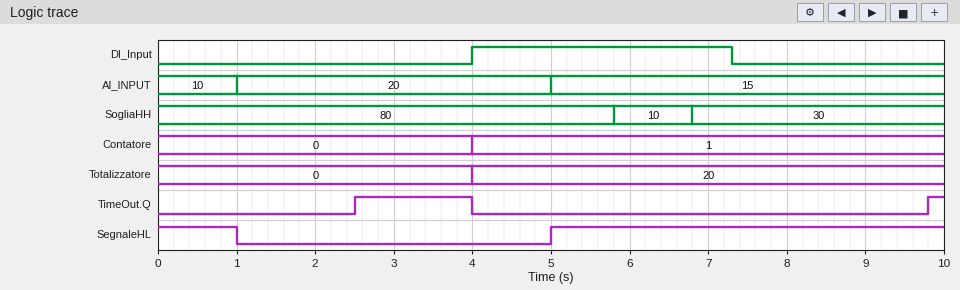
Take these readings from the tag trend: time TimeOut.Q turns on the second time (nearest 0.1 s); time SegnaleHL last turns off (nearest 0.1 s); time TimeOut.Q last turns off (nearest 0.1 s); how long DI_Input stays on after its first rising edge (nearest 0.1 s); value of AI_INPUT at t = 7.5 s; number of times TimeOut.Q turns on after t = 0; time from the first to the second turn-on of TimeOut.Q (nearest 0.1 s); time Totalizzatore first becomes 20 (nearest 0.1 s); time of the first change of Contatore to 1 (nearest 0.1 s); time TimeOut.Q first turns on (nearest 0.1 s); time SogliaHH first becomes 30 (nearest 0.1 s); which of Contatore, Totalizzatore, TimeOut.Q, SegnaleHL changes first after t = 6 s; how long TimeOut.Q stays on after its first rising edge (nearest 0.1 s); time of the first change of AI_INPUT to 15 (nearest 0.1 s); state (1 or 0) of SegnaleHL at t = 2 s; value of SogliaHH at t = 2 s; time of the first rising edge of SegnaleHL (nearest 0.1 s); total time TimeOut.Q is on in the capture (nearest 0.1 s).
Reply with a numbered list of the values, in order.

1. 9.8 s
2. 1.0 s
3. 4.0 s
4. 3.3 s
5. 15
6. 2
7. 7.3 s
8. 4.0 s
9. 4.0 s
10. 2.5 s
11. 6.8 s
12. TimeOut.Q
13. 1.5 s
14. 5.0 s
15. 0
16. 80
17. 5.0 s
18. 1.7 s
